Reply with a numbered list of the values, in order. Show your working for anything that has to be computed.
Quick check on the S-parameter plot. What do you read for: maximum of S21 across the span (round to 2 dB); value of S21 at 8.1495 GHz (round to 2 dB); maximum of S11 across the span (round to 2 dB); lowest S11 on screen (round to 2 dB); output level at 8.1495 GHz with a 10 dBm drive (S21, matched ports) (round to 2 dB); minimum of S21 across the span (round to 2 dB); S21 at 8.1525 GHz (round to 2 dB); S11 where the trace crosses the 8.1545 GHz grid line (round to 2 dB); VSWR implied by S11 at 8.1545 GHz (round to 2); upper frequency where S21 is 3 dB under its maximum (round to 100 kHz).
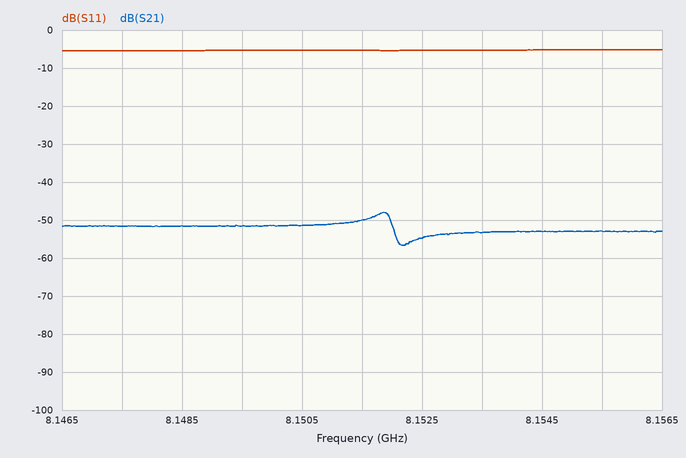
1. -48 dB
2. -52 dB
3. -6 dB
4. -6 dB
5. 10 dBm + (-52 dB) = -42 dBm
6. -56 dB
7. -54 dB
8. -6 dB
9. |Γ| = 10^(-6/20) = 0.5012; VSWR = (1 + 0.5012)/(1 − 0.5012) ≈ 3.01, so 4 to the nearest 2
10. 8.1520 GHz
